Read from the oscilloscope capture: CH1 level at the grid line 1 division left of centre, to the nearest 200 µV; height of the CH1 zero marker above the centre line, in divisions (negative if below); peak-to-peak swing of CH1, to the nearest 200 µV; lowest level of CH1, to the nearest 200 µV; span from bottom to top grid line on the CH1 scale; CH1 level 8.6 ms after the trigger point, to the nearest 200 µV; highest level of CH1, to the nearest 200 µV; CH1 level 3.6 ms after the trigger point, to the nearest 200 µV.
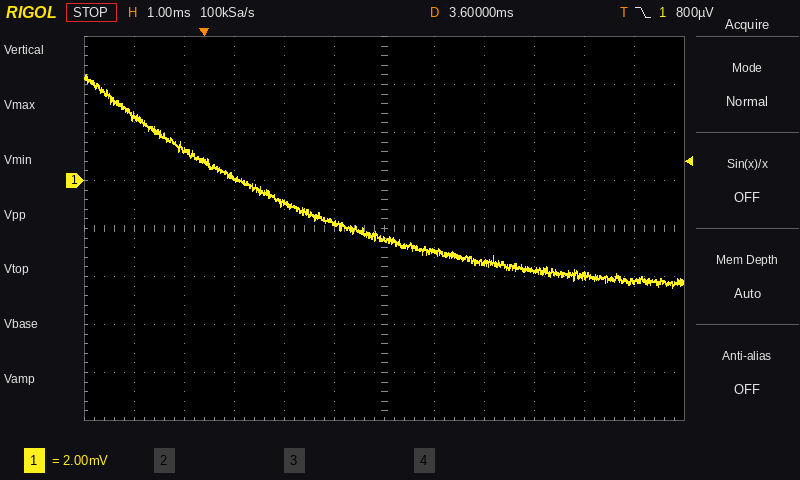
-1.8 mV
+1.0 div
8.8 mV
-4.4 mV
16 mV
-4.2 mV
4.4 mV
-2.4 mV
